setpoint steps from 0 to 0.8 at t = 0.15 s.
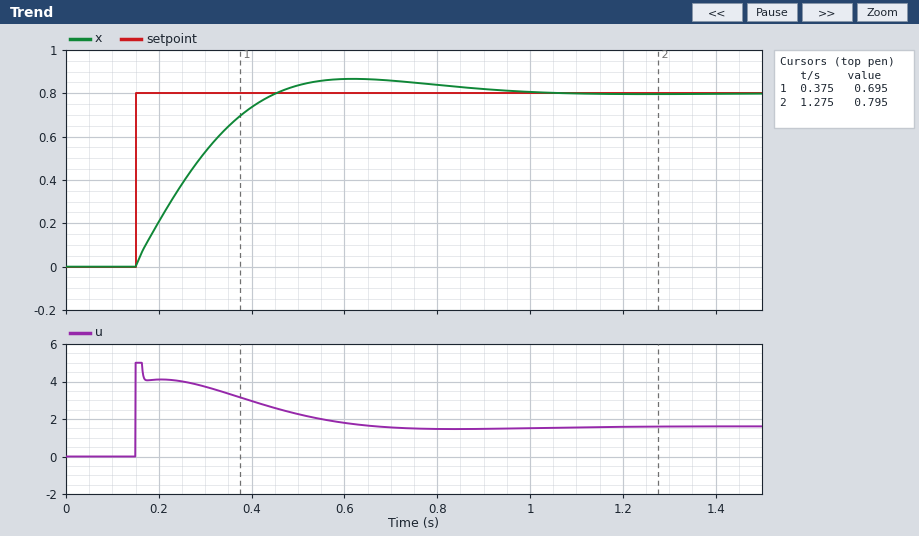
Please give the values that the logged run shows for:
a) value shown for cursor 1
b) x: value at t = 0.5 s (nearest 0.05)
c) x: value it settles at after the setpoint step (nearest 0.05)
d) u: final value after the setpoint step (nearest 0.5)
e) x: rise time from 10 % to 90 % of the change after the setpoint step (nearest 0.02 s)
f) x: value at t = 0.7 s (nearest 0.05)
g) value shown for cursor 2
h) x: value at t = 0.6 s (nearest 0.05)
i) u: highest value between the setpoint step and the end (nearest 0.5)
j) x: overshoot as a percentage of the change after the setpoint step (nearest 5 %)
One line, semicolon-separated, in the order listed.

0.695; 0.85; 0.80; 1.5; 0.22 s; 0.85; 0.795; 0.85; 5.0; 10 %
